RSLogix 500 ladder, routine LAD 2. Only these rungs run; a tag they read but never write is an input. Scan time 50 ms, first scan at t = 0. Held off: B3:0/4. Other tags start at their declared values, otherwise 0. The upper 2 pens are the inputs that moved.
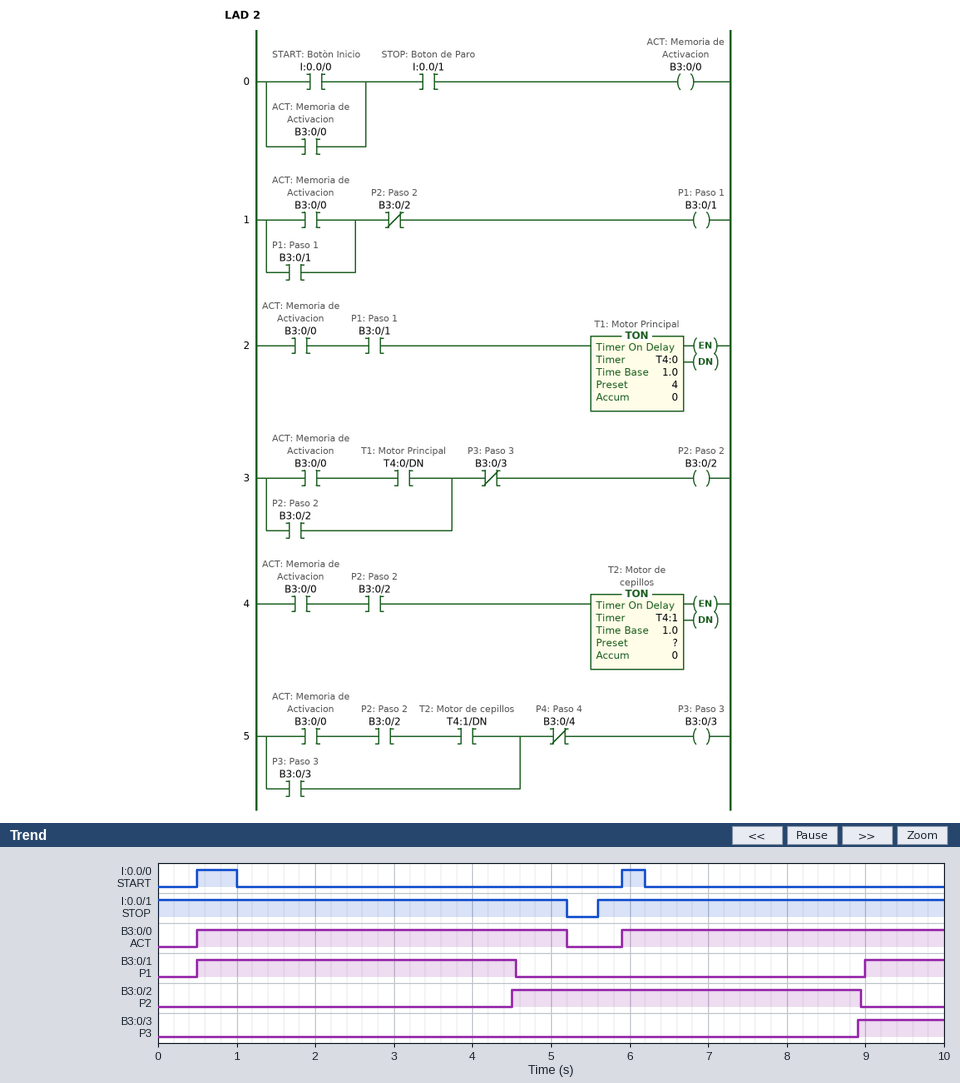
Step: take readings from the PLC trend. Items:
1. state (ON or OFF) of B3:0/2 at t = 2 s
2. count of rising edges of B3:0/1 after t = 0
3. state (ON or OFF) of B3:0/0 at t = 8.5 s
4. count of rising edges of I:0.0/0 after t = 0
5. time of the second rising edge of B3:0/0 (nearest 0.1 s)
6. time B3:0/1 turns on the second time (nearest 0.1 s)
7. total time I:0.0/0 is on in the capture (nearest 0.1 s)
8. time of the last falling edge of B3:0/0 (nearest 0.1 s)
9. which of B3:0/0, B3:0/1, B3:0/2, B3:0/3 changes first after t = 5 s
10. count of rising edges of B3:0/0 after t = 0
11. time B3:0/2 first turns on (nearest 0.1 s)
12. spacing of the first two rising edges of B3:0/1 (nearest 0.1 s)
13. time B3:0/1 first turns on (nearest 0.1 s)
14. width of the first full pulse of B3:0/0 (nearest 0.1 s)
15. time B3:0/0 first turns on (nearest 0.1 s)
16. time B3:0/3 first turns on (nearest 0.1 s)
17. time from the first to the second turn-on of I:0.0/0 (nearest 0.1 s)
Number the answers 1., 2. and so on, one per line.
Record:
1. OFF
2. 2
3. ON
4. 2
5. 5.9 s
6. 9.0 s
7. 0.8 s
8. 5.2 s
9. B3:0/0
10. 2
11. 4.5 s
12. 8.5 s
13. 0.5 s
14. 4.7 s
15. 0.5 s
16. 8.9 s
17. 5.4 s
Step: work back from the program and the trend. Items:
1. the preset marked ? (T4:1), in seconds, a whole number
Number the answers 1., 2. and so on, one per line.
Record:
1. 3 s
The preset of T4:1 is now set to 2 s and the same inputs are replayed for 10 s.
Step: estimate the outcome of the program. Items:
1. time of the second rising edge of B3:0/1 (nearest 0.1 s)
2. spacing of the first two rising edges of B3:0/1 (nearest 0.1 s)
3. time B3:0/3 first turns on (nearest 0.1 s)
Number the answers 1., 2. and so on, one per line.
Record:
1. 8.0 s
2. 7.5 s
3. 7.9 s
